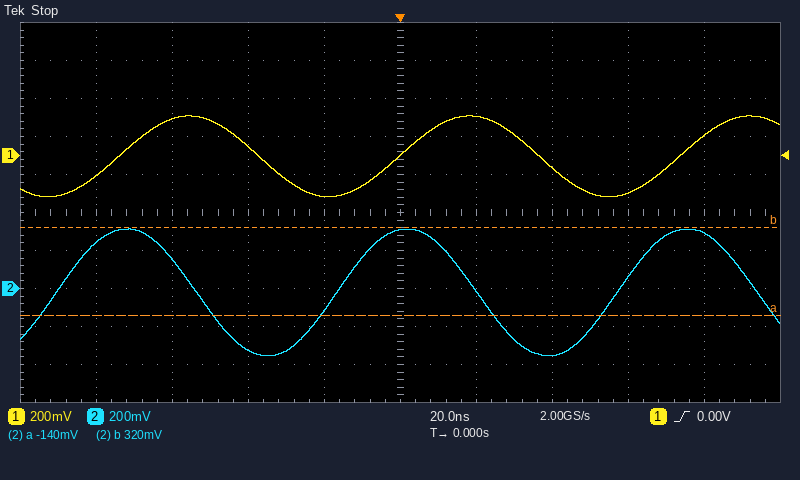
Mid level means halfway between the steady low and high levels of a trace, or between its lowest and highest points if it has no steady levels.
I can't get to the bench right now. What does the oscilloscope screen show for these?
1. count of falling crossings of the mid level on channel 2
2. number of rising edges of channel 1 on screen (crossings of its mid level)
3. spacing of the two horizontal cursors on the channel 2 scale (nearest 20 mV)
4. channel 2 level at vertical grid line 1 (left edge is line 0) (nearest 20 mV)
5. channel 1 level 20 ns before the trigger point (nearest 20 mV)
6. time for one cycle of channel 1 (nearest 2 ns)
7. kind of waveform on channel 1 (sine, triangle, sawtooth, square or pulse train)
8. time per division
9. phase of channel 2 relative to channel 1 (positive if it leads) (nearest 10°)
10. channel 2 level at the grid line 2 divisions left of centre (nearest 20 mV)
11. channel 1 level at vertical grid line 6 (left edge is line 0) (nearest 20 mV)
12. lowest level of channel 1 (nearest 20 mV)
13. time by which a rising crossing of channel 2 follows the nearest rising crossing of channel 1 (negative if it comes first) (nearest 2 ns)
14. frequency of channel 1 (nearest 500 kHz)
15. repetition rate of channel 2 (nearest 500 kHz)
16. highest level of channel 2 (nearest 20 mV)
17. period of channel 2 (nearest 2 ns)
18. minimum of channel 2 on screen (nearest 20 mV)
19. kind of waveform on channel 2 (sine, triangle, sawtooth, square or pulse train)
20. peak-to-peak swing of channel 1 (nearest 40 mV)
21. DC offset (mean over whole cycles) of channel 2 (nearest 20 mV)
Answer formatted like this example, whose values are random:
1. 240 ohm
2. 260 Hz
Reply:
1. 3
2. 3
3. 460 mV
4. 240 mV
5. -220 mV
6. 74 ns
7. sine
8. 20 ns
9. +80°
10. -320 mV
11. 200 mV
12. -220 mV
13. -16 ns
14. 13.5 MHz
15. 13.5 MHz
16. 320 mV
17. 74 ns
18. -360 mV
19. sine
20. 440 mV
21. -20 mV
